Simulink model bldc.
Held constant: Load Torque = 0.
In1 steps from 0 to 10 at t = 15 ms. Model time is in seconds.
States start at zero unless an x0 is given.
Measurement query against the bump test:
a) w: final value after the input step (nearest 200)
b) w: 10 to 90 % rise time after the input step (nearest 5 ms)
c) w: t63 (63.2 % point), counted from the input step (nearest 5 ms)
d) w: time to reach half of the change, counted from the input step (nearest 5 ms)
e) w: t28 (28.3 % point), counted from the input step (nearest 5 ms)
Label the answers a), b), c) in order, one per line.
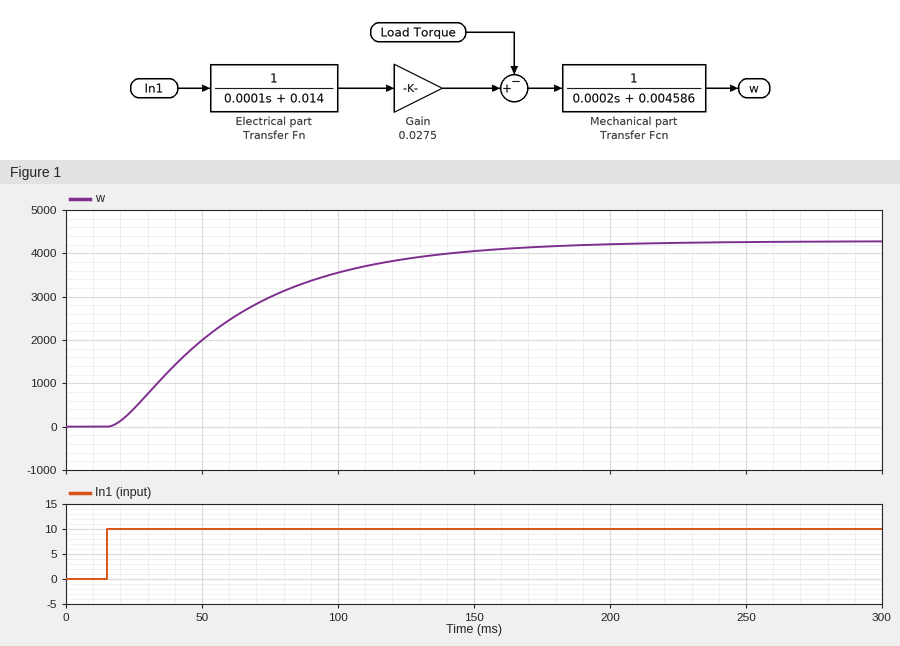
a) 4200
b) 100 ms
c) 50 ms
d) 40 ms
e) 20 ms
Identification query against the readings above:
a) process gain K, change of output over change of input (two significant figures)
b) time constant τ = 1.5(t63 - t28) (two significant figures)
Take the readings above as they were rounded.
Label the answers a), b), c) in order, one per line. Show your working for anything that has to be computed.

a) (4200 - 0) / 10 = 420
b) 1.5 × (50 - 20) = 45 ms
